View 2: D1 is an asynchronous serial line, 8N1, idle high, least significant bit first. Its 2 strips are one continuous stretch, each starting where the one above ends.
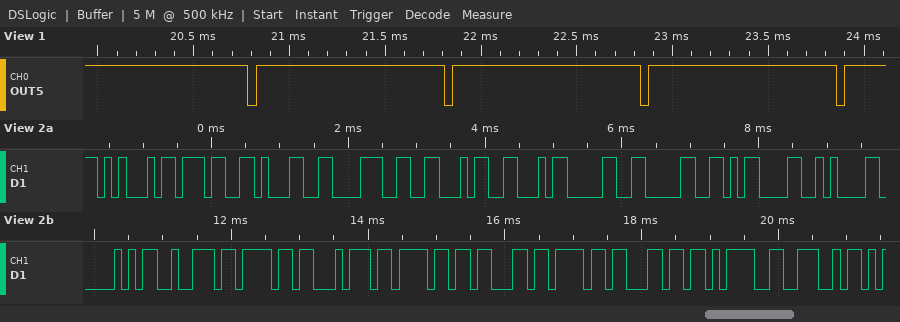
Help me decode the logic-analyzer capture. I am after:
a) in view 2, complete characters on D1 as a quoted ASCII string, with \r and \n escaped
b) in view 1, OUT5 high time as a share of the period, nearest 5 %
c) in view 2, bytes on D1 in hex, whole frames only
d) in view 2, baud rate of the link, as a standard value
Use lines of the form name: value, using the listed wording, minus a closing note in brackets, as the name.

in view 2, complete characters on D1 as a quoted ASCII string, with \r and \n escaped: "E718FF00\r\nProtocol=N"
in view 1, OUT5 high time as a share of the period, nearest 5 %: 95 %
in view 2, bytes on D1 in hex, whole frames only: 45 37 31 38 46 46 30 30 0D 0A 50 72 6F 74 6F 63 6F 6C 3D 4E
in view 2, baud rate of the link, as a standard value: 9600 baud
